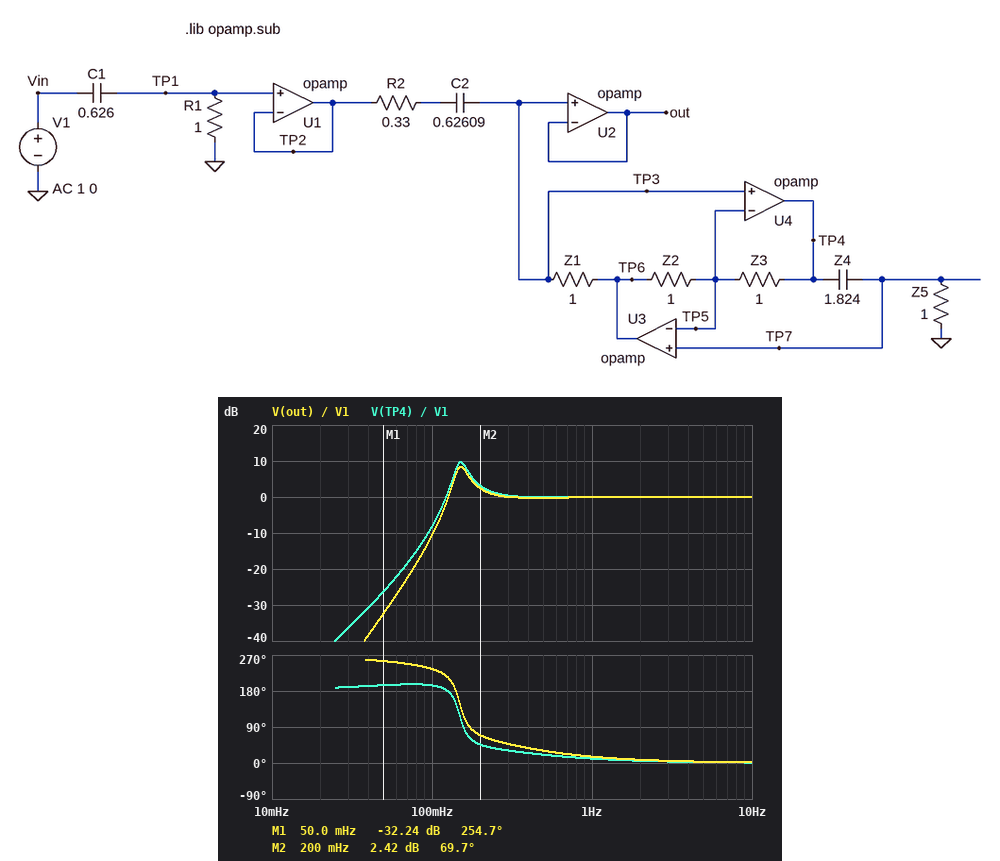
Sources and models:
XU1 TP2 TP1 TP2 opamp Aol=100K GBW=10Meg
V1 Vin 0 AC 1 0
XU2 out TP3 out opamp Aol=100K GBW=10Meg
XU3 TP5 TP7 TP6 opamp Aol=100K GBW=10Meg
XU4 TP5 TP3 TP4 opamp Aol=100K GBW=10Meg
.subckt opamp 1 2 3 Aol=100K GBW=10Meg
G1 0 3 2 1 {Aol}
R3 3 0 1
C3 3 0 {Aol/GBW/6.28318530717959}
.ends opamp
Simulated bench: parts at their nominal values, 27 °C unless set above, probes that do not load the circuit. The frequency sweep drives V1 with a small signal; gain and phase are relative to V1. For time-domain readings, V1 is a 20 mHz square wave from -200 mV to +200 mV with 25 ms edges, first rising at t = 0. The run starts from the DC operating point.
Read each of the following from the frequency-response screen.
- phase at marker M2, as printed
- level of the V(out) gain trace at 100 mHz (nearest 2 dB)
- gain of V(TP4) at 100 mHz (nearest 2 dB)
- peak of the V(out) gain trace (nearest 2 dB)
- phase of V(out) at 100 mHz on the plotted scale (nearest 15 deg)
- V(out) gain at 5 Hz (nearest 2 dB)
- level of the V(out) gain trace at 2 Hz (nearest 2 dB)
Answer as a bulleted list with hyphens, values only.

- 69.7 deg
- -10 dB
- -8 dB
- 8 dB
- 240 deg
- 0 dB
- 0 dB
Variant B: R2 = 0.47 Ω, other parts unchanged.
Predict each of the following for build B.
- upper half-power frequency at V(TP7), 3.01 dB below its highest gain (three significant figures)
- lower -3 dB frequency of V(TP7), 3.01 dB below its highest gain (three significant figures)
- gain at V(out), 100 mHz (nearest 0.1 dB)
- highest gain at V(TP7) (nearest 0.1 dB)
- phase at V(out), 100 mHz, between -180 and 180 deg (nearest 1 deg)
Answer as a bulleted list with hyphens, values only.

- 192 mHz
- 137 mHz
- -10.9 dB
- 5.5 dB
- -130 deg
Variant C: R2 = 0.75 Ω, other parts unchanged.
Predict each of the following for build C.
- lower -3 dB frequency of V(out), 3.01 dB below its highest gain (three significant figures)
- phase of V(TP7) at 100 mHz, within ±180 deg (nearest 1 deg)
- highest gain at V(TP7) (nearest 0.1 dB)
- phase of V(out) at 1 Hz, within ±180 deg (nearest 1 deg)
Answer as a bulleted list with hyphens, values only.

- 135 mHz
- -140 deg
- 1.9 dB
- 18 deg
